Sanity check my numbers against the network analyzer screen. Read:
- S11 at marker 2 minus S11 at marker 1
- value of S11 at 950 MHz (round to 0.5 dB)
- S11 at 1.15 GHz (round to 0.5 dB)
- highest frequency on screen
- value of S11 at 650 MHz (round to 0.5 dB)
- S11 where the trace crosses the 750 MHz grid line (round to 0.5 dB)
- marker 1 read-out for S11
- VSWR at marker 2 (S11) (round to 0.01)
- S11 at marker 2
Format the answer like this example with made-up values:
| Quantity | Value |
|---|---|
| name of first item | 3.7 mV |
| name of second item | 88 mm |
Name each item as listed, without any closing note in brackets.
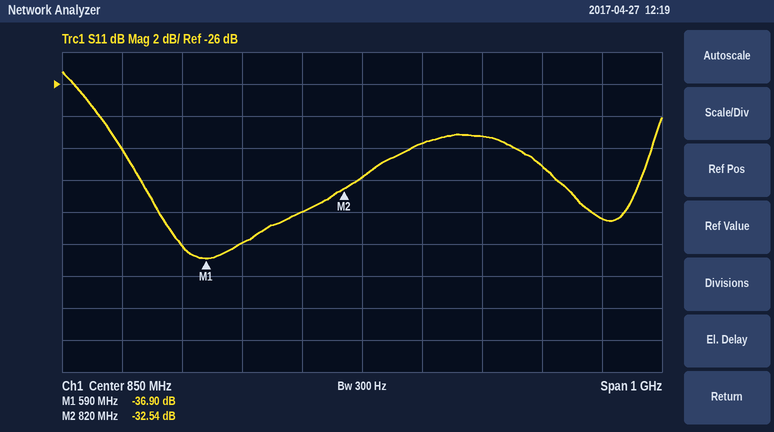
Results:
| Quantity | Value |
|---|---|
| S11 at marker 2 minus S11 at marker 1 | 4.36 dB |
| value of S11 at 950 MHz | -29.5 dB |
| S11 at 1.15 GHz | -31.0 dB |
| highest frequency on screen | 1.35 GHz |
| value of S11 at 650 MHz | -36.0 dB |
| S11 where the trace crosses the 750 MHz grid line | -34.0 dB |
| marker 1 read-out for S11 | -36.90 dB |
| VSWR at marker 2 (S11) | 1.05 |
| S11 at marker 2 | -32.54 dB |
